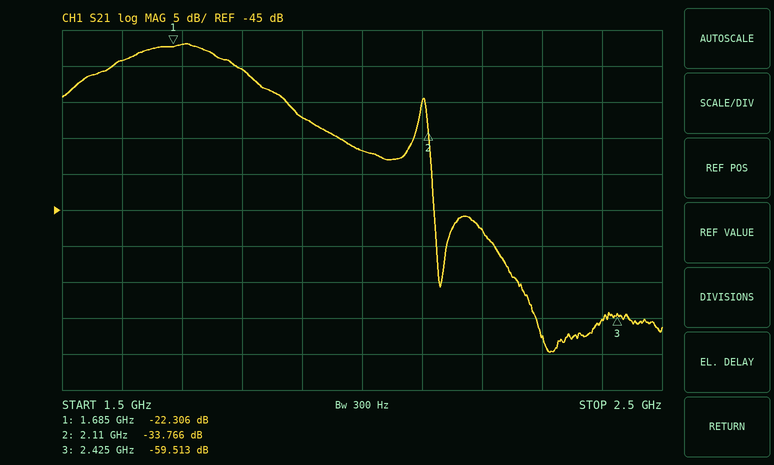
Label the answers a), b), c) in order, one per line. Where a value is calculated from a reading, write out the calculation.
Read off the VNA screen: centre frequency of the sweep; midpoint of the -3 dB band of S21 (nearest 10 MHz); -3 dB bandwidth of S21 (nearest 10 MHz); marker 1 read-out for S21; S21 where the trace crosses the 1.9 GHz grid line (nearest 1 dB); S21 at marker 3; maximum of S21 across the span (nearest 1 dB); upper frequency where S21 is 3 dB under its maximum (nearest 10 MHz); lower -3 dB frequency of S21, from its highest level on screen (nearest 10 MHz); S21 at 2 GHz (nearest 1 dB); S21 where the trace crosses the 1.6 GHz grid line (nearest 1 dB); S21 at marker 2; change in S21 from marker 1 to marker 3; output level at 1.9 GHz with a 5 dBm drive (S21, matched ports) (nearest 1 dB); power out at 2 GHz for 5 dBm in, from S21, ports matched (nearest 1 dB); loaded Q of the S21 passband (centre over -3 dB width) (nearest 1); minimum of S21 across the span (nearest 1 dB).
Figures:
a) 2 GHz
b) 1.69 GHz
c) 1.79 GHz − 1.59 GHz = 200 MHz
d) -22.306 dB
e) -32 dB
f) -59.513 dB
g) -22 dB
h) 1.79 GHz
i) 1.59 GHz
j) -37 dB
k) -24 dB
l) -33.766 dB
m) -59.513 − (-22.306) = -37.207 dB
n) 5 dBm + (-32 dB) = -27 dBm
o) 5 dBm + (-37 dB) = -32 dBm
p) 1.69 GHz / 200 MHz ≈ 8
q) -65 dB
